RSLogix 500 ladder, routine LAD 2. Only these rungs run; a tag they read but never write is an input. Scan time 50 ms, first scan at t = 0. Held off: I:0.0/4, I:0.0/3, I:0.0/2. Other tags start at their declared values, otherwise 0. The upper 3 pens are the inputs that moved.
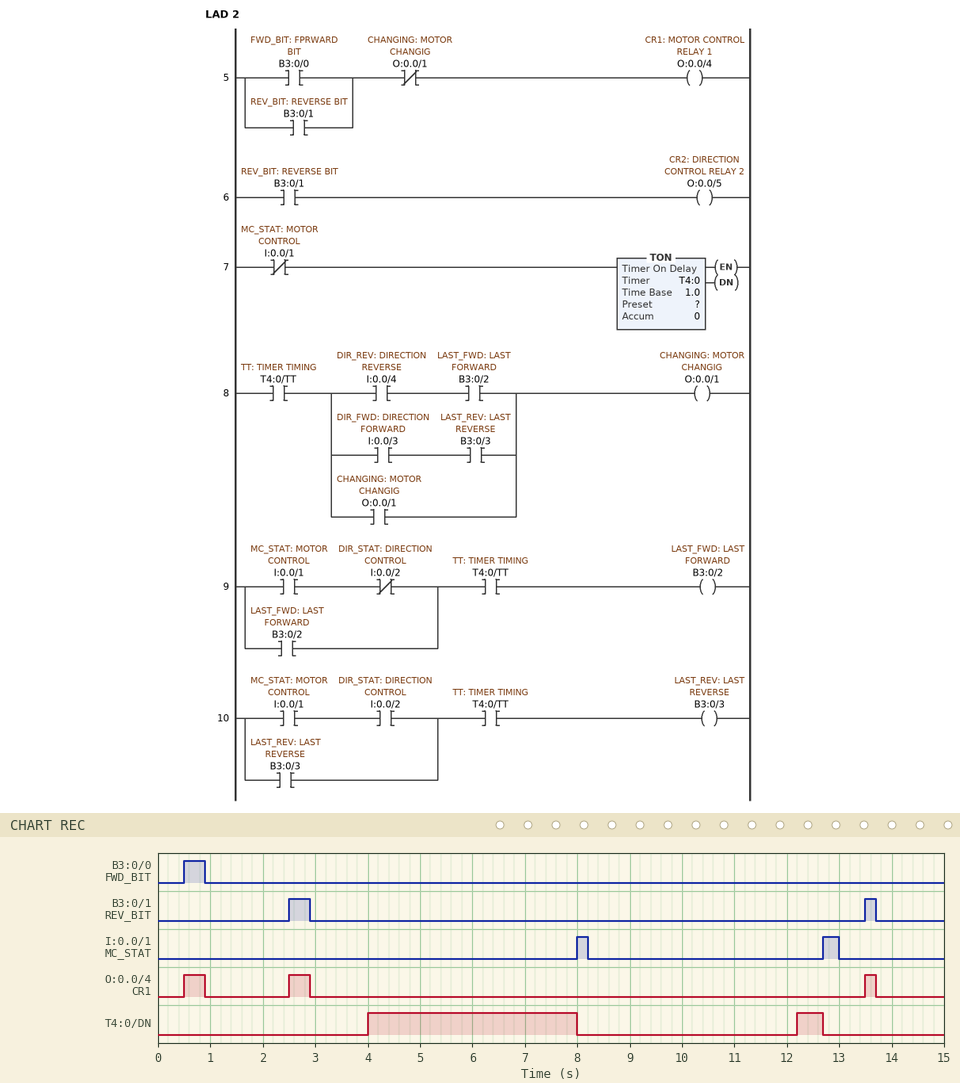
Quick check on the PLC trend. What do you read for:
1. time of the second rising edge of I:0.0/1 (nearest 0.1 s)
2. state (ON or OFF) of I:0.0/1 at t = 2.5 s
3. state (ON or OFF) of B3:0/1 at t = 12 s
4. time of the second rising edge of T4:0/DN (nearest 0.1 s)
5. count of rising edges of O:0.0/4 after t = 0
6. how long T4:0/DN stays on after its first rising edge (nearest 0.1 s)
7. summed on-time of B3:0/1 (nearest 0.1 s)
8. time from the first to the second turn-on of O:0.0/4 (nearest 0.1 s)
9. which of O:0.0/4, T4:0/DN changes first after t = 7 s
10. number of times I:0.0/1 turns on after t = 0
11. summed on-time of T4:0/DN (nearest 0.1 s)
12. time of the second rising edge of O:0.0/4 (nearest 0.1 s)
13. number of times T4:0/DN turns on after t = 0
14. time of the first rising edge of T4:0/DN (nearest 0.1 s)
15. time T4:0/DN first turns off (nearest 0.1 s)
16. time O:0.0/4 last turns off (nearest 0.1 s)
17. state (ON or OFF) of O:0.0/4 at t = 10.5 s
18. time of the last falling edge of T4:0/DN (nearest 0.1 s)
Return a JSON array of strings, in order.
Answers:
["12.7 s", "OFF", "OFF", "12.2 s", "3", "4.0 s", "0.6 s", "2.0 s", "T4:0/DN", "2", "4.5 s", "2.5 s", "2", "4.0 s", "8.0 s", "13.7 s", "OFF", "12.7 s"]
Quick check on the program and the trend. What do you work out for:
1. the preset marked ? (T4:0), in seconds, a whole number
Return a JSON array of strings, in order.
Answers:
["4 s"]
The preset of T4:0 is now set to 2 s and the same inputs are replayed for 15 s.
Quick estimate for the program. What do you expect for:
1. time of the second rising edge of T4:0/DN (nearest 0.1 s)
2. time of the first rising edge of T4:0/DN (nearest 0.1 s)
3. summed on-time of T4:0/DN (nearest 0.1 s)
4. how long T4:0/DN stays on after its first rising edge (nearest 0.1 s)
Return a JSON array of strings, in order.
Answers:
["10.2 s", "2.0 s", "8.5 s", "6.0 s"]
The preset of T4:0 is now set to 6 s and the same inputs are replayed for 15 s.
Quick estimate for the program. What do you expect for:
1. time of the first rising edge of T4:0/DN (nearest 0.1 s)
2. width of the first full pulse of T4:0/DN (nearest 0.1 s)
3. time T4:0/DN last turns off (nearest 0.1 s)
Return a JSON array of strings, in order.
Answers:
["6.0 s", "2.0 s", "8.0 s"]
